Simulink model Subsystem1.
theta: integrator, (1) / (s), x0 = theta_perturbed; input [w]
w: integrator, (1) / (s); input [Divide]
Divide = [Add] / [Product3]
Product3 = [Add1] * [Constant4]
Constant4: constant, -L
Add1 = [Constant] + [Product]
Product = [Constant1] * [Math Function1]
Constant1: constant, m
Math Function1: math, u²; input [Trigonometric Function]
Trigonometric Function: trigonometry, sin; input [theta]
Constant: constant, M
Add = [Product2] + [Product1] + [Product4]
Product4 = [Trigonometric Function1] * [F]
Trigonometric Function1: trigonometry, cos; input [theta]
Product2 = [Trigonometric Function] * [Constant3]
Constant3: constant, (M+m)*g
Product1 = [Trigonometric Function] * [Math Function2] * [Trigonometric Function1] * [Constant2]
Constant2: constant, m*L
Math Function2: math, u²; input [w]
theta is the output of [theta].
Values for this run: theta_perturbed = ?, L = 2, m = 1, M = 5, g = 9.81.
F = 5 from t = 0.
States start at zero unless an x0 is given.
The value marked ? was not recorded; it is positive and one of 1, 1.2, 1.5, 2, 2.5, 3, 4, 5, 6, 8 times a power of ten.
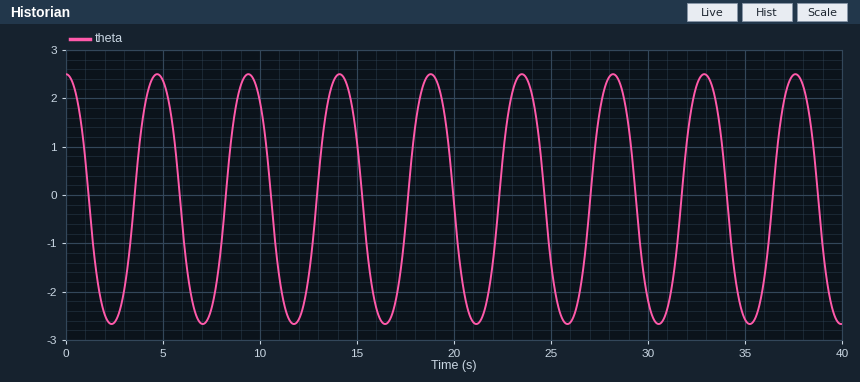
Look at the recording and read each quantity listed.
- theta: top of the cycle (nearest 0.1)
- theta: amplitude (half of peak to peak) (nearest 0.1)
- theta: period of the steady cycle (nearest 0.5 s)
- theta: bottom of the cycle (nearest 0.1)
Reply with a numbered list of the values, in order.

1. 2.5
2. 2.6
3. 4.5 s
4. -2.7
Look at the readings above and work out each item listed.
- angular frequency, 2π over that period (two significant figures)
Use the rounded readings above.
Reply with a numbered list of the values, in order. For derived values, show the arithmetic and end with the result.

1. 2π / 4.5 = 1.4 rad/s
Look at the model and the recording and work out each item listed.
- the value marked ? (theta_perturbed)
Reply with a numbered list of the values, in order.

1. 2.5
